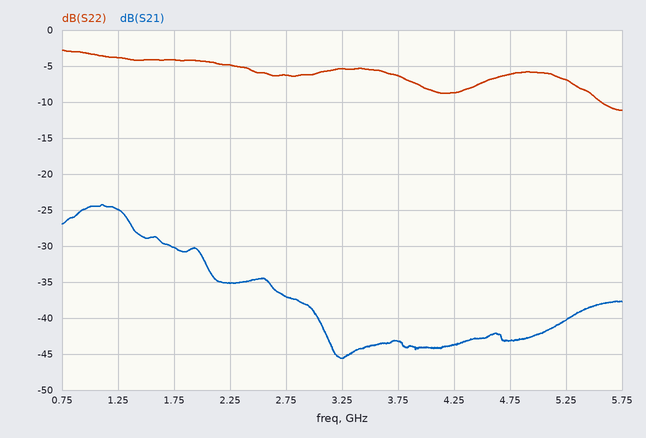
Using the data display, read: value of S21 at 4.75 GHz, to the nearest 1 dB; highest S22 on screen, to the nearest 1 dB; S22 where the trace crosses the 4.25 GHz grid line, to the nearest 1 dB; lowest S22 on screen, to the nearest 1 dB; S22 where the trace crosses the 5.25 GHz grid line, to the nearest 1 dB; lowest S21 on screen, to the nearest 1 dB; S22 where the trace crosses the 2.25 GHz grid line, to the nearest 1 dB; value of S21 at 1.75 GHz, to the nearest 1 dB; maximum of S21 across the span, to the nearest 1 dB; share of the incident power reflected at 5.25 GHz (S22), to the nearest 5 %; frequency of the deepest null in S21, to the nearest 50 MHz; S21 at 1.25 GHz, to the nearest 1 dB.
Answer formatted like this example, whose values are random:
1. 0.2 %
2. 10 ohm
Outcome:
1. -43 dB
2. -3 dB
3. -9 dB
4. -11 dB
5. -7 dB
6. -46 dB
7. -5 dB
8. -30 dB
9. -24 dB
10. 20 %
11. 3.25 GHz
12. -25 dB
